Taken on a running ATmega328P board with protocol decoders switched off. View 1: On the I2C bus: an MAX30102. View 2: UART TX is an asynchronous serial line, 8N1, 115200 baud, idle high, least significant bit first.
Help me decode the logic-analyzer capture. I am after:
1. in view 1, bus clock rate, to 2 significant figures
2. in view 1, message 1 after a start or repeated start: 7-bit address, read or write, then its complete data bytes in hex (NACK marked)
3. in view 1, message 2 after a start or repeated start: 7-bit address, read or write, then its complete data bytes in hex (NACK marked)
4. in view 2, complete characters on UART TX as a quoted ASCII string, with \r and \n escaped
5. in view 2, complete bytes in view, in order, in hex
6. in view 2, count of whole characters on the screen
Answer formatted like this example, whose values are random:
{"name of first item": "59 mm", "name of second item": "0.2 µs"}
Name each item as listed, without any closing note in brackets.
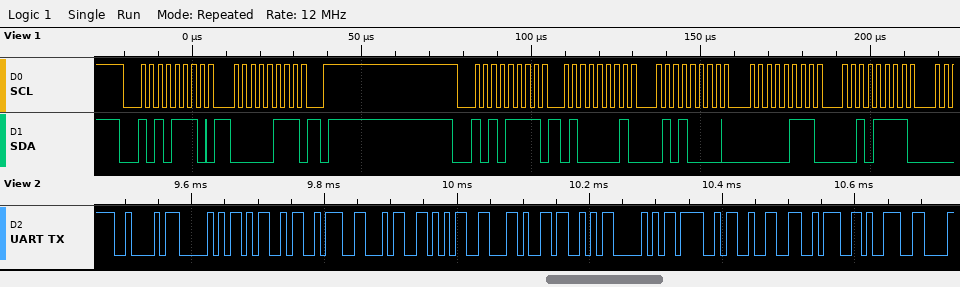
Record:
{"in view 1, bus clock rate, to 2 significant figures": "400 kHz", "in view 1, message 1 after a start or repeated start: 7-bit address, read or write, then its complete data bytes in hex": "0x57 write: 07", "in view 1, message 2 after a start or repeated start: 7-bit address, read or write, then its complete data bytes in hex": "0x57 read: 41 50 07 2F", "in view 2, complete characters on UART TX as a quoted ASCII string, with \\r and \\n escaped": "\"BPM:45,SPO2:9\"", "in view 2, complete bytes in view, in order, in hex": "42 50 4D 3A 34 35 2C 53 50 4F 32 3A 39", "in view 2, count of whole characters on the screen": "13"}
